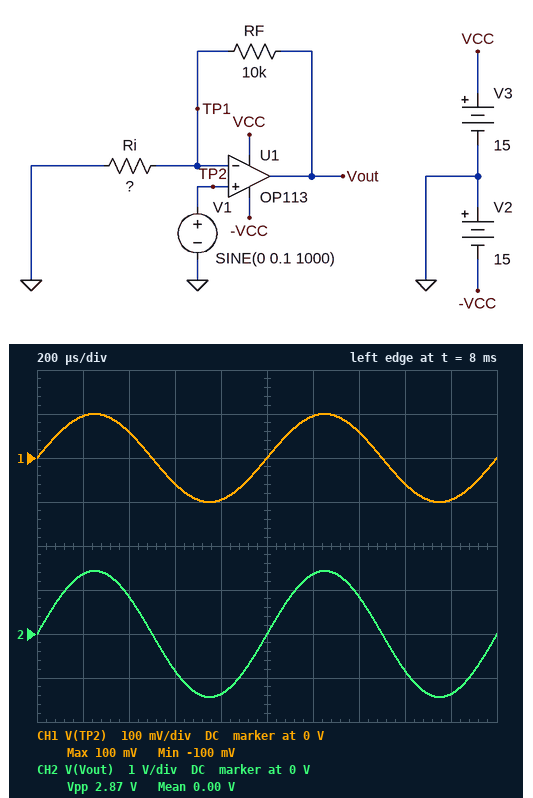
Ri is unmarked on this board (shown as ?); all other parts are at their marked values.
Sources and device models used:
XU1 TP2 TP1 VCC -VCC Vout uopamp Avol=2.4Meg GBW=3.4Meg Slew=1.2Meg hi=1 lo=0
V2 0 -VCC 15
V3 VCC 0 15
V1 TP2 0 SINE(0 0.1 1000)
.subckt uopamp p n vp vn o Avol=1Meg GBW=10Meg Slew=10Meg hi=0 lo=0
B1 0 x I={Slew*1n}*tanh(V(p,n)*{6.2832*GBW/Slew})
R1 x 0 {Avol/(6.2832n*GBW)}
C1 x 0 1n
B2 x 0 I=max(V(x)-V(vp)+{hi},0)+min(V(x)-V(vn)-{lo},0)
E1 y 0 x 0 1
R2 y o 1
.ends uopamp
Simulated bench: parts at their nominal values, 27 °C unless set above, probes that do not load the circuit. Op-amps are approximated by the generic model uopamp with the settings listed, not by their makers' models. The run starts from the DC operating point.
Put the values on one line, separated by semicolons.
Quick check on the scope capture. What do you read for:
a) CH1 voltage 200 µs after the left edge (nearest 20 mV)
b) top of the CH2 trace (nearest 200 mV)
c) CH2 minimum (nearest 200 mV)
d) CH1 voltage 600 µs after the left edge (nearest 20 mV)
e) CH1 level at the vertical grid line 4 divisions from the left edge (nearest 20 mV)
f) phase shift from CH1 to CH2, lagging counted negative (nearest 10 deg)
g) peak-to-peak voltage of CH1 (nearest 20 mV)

100 mV; 1.4 V; -1.4 V; -60 mV; -100 mV; 0 deg; 200 mV
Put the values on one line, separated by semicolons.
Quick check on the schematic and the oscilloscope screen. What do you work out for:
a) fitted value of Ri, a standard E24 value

750 Ω
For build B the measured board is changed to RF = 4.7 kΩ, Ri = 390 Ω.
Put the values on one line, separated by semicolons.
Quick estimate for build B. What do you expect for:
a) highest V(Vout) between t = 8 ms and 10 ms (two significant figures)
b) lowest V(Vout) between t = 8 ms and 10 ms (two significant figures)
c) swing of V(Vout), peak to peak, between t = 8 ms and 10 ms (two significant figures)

1.3 V; -1.3 V; 2.6 V
